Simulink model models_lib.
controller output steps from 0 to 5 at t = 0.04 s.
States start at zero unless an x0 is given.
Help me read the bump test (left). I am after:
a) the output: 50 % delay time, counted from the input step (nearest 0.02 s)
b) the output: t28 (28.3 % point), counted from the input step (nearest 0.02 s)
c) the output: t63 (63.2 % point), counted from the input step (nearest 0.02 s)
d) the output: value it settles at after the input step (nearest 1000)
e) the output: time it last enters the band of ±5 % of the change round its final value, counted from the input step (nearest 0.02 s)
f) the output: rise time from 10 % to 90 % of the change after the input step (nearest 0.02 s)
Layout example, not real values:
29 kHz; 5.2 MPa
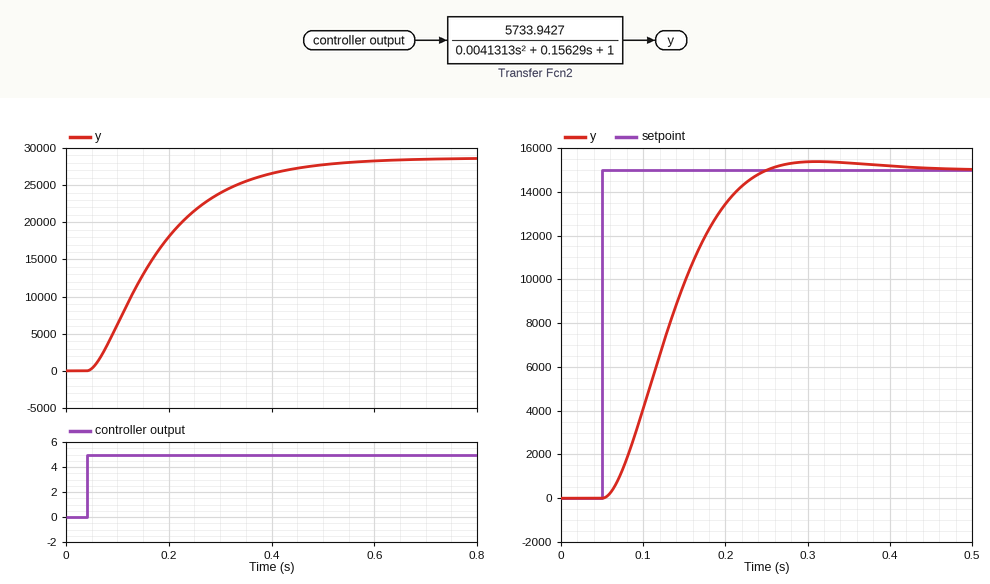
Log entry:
0.12 s; 0.08 s; 0.16 s; 29000; 0.40 s; 0.28 s
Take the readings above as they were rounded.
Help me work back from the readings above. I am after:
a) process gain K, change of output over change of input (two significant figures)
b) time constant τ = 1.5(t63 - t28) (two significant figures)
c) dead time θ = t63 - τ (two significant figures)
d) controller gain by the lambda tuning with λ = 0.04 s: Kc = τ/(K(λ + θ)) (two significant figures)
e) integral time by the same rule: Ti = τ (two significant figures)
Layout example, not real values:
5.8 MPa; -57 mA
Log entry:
5800; 0.12 s; 0.040 s; 0.00026; 0.12 s
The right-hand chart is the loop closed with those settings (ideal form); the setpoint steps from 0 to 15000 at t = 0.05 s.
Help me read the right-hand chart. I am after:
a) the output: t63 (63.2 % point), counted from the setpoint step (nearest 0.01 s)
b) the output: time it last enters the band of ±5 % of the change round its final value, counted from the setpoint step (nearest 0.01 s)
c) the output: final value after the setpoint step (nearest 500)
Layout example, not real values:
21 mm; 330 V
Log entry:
0.10 s; 0.17 s; 15000
